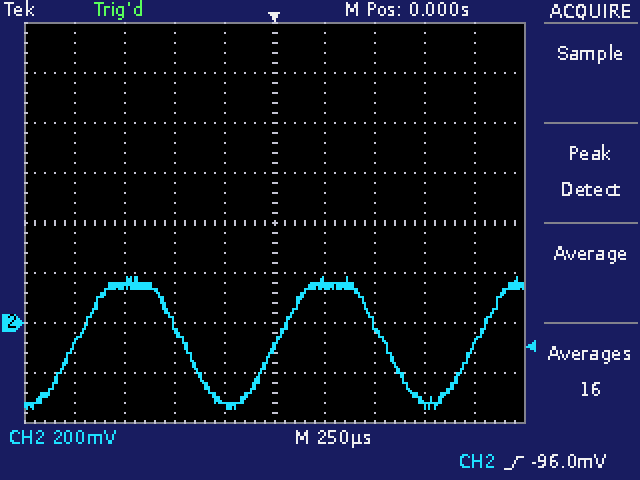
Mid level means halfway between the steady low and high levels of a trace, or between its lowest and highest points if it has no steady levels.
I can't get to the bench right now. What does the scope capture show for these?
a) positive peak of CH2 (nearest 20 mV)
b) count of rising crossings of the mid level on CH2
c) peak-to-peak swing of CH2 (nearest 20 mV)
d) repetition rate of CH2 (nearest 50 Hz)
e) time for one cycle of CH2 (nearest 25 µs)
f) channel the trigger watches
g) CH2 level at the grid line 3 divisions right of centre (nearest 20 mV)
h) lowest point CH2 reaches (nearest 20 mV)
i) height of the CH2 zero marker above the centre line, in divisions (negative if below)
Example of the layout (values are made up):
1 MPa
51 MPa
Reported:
180 mV
3
520 mV
1.00 kHz
1.000 ms
CH2
-320 mV
-340 mV
-2.0 div
